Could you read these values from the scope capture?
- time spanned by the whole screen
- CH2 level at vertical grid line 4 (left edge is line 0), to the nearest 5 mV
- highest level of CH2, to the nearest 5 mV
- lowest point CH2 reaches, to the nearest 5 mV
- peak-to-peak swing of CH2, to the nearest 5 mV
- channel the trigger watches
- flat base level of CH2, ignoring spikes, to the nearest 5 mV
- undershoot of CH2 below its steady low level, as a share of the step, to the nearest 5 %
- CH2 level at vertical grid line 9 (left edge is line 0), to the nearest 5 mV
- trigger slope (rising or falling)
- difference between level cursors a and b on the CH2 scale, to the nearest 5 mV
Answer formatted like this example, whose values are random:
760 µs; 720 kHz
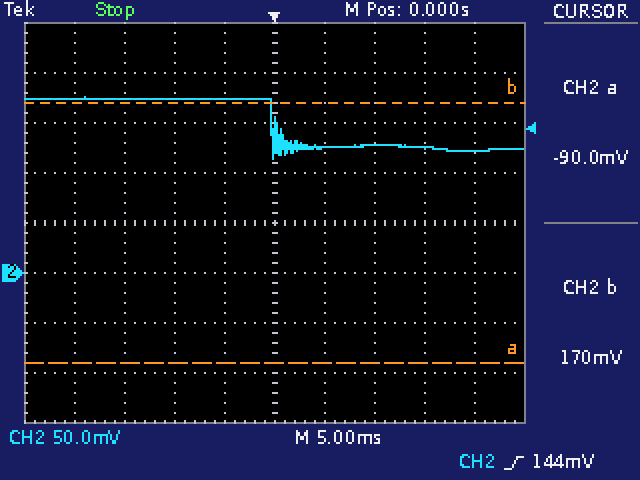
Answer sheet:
50 ms; 175 mV; 175 mV; 115 mV; 60 mV; CH2; 125 mV; 25 %; 120 mV; rising; 260 mV
